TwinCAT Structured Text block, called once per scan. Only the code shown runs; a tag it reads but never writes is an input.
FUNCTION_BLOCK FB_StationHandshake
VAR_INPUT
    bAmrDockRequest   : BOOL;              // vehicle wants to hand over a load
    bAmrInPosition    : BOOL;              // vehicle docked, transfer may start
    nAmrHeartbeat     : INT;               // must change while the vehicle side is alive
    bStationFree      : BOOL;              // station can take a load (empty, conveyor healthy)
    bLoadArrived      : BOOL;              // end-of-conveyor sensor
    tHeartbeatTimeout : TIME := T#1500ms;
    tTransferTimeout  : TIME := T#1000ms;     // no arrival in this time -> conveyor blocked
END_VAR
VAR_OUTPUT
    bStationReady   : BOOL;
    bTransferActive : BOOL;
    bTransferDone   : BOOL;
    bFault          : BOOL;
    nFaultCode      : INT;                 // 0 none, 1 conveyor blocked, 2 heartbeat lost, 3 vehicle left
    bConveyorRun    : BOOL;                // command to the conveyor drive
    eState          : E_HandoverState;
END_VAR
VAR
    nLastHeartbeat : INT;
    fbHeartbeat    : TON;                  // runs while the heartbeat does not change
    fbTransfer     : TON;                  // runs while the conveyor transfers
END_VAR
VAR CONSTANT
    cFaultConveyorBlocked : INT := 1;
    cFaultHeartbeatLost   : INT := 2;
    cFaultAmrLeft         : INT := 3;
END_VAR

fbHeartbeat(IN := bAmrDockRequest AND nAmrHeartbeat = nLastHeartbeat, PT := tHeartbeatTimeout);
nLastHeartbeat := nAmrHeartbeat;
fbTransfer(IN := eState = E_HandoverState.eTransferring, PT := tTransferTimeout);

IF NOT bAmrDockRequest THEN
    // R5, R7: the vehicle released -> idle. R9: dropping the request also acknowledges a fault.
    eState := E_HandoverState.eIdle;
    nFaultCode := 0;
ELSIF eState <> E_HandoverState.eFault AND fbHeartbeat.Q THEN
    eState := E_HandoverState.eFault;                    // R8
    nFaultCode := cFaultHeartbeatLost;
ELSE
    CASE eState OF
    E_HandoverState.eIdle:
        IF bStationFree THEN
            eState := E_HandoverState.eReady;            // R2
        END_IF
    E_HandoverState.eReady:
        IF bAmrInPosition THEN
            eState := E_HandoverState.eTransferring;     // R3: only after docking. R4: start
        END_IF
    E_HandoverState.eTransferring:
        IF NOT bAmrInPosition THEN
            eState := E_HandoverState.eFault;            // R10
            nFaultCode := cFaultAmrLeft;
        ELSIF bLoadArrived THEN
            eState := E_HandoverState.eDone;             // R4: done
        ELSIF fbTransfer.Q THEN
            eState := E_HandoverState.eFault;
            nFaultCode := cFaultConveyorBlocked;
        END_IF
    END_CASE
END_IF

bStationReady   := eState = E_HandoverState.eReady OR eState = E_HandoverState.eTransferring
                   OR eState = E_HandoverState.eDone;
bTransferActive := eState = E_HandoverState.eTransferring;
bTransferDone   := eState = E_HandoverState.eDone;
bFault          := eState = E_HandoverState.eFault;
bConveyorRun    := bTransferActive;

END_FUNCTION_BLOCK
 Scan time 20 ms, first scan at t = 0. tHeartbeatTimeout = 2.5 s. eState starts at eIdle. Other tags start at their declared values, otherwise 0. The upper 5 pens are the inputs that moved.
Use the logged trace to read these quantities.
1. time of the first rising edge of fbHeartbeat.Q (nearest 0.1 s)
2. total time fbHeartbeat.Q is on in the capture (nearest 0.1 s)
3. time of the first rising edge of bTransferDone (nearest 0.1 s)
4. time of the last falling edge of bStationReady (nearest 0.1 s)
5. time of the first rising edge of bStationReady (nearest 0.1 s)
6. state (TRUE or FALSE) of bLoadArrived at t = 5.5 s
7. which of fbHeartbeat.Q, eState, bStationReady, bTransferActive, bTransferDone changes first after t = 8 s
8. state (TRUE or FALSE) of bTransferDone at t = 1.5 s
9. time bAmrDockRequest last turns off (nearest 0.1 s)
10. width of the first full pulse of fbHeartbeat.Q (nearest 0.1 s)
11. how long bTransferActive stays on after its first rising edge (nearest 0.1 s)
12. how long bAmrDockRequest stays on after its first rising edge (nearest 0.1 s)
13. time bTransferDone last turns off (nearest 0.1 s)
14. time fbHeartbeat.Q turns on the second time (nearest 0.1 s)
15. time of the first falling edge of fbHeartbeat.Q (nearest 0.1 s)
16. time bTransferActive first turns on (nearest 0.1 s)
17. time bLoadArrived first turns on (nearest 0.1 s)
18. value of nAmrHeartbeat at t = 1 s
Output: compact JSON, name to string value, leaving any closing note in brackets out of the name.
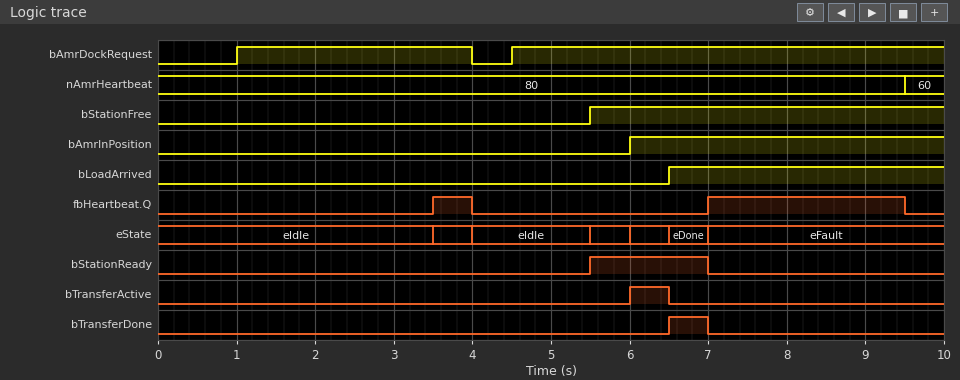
{"time of the first rising edge of fbHeartbeat.Q": "3.5 s", "total time fbHeartbeat.Q is on in the capture": "3.0 s", "time of the first rising edge of bTransferDone": "6.5 s", "time of the last falling edge of bStationReady": "7.0 s", "time of the first rising edge of bStationReady": "5.5 s", "state (TRUE or FALSE) of bLoadArrived at t = 5.5 s": "FALSE", "which of fbHeartbeat.Q, eState, bStationReady, bTransferActive, bTransferDone changes first after t = 8 s": "fbHeartbeat.Q", "state (TRUE or FALSE) of bTransferDone at t = 1.5 s": "FALSE", "time bAmrDockRequest last turns off": "4.0 s", "width of the first full pulse of fbHeartbeat.Q": "0.5 s", "how long bTransferActive stays on after its first rising edge": "0.5 s", "how long bAmrDockRequest stays on after its first rising edge": "3.0 s", "time bTransferDone last turns off": "7.0 s", "time fbHeartbeat.Q turns on the second time": "7.0 s", "time of the first falling edge of fbHeartbeat.Q": "4.0 s", "time bTransferActive first turns on": "6.0 s", "time bLoadArrived first turns on": "6.5 s", "value of nAmrHeartbeat at t = 1 s": "80"}
